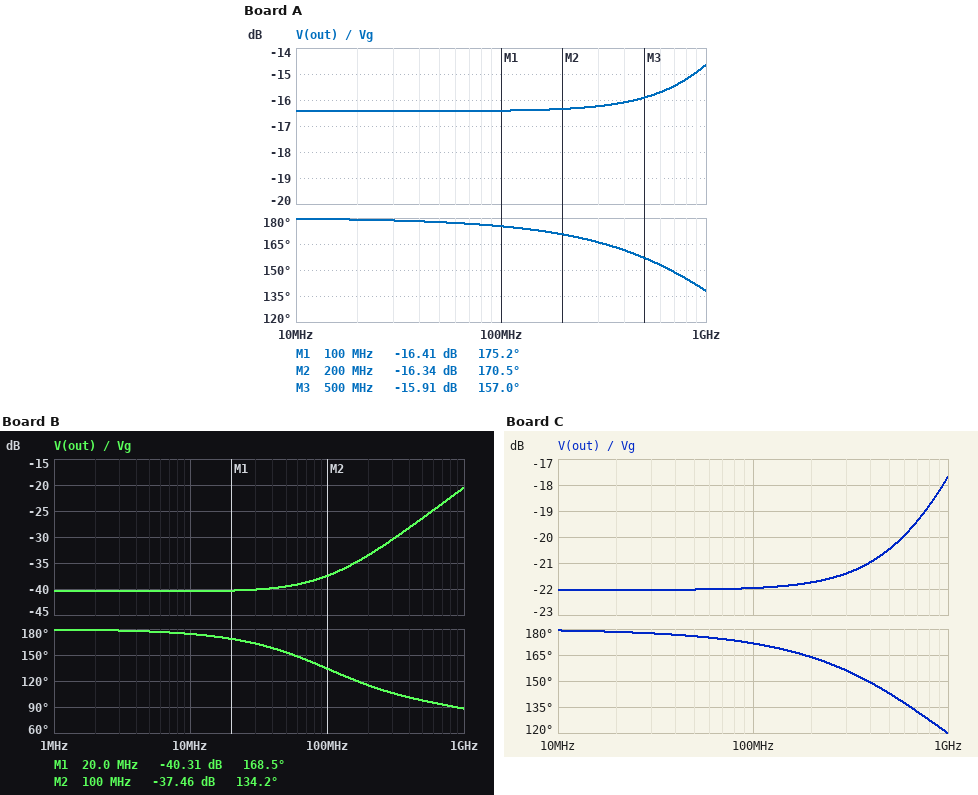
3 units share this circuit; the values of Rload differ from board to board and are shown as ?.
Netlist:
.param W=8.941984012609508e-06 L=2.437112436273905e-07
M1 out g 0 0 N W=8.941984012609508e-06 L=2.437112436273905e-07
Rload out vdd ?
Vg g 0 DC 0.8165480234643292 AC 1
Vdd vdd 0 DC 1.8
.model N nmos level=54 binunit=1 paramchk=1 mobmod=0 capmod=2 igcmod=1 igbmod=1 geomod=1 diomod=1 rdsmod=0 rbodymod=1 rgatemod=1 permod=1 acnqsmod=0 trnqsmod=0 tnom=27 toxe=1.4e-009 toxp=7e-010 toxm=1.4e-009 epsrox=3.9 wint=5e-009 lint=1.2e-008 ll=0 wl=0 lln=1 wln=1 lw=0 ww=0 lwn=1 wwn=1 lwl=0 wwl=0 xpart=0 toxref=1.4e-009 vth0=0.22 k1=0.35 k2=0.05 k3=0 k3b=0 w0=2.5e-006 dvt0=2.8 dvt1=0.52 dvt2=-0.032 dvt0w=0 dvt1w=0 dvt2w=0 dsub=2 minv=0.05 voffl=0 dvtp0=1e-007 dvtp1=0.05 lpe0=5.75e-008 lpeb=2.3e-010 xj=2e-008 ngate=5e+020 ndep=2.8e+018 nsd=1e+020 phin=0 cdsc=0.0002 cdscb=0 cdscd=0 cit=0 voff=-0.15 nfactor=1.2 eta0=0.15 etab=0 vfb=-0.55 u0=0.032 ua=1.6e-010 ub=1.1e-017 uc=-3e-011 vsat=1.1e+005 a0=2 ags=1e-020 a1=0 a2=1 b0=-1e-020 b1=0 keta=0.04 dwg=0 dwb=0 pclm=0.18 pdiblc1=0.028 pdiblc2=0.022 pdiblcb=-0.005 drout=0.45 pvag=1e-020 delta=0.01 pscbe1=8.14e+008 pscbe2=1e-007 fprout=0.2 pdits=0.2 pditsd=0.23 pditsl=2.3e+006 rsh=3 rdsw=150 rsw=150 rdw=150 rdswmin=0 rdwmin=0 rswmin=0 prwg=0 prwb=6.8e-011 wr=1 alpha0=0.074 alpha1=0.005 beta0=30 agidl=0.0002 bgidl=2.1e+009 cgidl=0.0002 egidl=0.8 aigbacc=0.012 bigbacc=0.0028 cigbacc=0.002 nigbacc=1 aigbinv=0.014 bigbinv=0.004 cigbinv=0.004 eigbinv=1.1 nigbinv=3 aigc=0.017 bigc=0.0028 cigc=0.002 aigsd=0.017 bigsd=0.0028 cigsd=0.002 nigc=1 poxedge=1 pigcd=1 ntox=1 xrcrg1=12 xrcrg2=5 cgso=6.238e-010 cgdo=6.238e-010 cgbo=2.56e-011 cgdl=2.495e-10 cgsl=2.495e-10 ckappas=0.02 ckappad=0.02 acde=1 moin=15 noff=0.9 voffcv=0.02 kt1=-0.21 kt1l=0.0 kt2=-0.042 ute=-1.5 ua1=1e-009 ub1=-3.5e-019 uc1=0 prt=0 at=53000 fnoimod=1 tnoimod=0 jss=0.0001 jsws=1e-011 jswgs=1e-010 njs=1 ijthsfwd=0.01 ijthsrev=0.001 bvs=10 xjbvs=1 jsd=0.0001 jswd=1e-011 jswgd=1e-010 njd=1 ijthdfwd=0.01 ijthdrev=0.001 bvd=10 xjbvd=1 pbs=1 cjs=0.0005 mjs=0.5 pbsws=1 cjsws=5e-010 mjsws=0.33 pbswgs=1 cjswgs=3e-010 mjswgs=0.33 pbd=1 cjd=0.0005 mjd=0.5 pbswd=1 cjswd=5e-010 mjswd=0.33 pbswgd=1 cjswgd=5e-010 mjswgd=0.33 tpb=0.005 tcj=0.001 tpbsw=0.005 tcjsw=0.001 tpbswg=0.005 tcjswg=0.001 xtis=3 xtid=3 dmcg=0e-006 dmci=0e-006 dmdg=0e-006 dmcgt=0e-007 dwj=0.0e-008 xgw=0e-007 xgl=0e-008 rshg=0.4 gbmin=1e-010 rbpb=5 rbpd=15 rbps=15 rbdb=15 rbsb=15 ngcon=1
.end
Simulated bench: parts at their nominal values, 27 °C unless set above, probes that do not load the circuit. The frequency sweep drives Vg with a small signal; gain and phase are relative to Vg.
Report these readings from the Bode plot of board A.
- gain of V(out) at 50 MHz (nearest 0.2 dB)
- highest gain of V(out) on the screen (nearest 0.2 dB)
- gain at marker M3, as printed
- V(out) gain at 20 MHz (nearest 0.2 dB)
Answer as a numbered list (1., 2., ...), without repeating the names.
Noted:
1. -16.4 dB
2. -14.6 dB
3. -15.91 dB
4. -16.4 dB
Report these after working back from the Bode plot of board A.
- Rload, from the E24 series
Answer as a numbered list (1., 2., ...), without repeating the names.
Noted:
1. 4.3 kΩ
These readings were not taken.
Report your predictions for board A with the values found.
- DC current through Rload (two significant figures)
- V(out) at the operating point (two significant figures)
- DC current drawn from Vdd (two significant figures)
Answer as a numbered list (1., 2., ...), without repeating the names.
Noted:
1. 380 µA
2. 150 mV
3. 380 µA
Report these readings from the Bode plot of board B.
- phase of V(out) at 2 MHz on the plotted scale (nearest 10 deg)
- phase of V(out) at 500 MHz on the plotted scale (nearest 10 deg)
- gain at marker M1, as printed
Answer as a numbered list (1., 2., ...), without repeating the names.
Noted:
1. 180 deg
2. 100 deg
3. -40.31 dB
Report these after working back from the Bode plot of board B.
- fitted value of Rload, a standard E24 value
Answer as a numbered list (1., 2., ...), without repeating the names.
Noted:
1. 33 kΩ
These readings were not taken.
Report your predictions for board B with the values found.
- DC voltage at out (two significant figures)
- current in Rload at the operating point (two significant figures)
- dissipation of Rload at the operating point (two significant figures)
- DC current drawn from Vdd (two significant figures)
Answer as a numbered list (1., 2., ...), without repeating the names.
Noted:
1. 17 mV
2. 54 µA
3. 96 µW
4. 54 µA
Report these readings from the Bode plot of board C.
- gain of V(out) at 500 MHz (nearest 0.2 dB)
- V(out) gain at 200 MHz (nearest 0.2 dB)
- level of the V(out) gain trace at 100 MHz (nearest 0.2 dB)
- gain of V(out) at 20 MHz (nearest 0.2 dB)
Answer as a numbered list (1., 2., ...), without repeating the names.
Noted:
1. -20.4 dB
2. -21.8 dB
3. -22.0 dB
4. -22.0 dB
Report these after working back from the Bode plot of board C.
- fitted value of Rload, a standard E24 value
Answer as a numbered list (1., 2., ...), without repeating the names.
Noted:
1. 6.2 kΩ
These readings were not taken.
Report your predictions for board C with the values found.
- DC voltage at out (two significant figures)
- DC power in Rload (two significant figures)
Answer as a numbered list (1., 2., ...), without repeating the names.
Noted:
1. 98 mV
2. 470 µW
